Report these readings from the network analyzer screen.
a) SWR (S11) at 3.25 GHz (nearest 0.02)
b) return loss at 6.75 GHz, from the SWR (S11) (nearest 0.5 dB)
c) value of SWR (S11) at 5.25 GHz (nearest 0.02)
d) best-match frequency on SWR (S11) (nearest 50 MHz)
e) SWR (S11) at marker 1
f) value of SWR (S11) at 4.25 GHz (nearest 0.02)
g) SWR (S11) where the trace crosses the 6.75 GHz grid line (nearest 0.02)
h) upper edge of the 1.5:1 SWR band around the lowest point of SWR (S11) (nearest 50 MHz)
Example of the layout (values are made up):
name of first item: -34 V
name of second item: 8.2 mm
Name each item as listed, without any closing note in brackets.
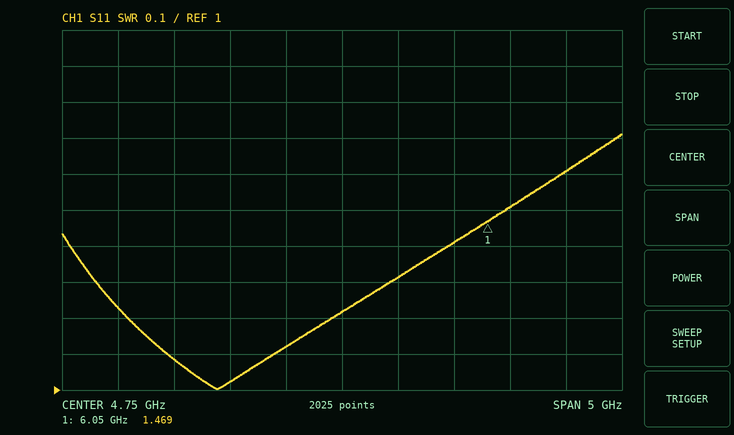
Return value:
SWR (S11) at 3.25 GHz: 1.08
return loss at 6.75 GHz, from the SWR (S11): 12.5 dB
value of SWR (S11) at 5.25 GHz: 1.32
best-match frequency on SWR (S11): 3.65 GHz
SWR (S11) at marker 1: 1.469
value of SWR (S11) at 4.25 GHz: 1.12
SWR (S11) where the trace crosses the 6.75 GHz grid line: 1.60
upper edge of the 1.5:1 SWR band around the lowest point of SWR (S11): 6.20 GHz
